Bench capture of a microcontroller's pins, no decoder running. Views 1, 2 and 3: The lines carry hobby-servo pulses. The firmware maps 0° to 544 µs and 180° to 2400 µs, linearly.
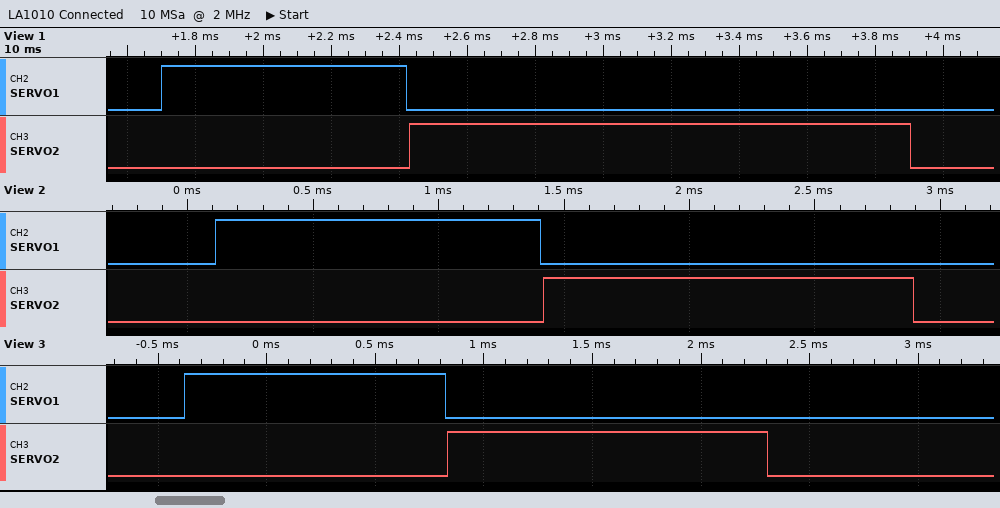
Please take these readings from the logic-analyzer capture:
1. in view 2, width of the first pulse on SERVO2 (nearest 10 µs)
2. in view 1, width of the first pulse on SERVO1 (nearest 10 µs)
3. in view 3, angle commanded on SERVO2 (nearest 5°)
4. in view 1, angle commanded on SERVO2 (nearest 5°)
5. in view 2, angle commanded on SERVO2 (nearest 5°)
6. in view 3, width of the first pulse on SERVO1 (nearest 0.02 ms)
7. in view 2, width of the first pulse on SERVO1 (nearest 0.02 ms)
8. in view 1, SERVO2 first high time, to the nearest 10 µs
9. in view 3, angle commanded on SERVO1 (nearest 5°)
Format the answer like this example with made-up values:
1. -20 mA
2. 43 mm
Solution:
1. 1470 µs
2. 720 µs
3. 90°
4. 90°
5. 90°
6. 1.20 ms
7. 1.30 ms
8. 1470 µs
9. 65°
